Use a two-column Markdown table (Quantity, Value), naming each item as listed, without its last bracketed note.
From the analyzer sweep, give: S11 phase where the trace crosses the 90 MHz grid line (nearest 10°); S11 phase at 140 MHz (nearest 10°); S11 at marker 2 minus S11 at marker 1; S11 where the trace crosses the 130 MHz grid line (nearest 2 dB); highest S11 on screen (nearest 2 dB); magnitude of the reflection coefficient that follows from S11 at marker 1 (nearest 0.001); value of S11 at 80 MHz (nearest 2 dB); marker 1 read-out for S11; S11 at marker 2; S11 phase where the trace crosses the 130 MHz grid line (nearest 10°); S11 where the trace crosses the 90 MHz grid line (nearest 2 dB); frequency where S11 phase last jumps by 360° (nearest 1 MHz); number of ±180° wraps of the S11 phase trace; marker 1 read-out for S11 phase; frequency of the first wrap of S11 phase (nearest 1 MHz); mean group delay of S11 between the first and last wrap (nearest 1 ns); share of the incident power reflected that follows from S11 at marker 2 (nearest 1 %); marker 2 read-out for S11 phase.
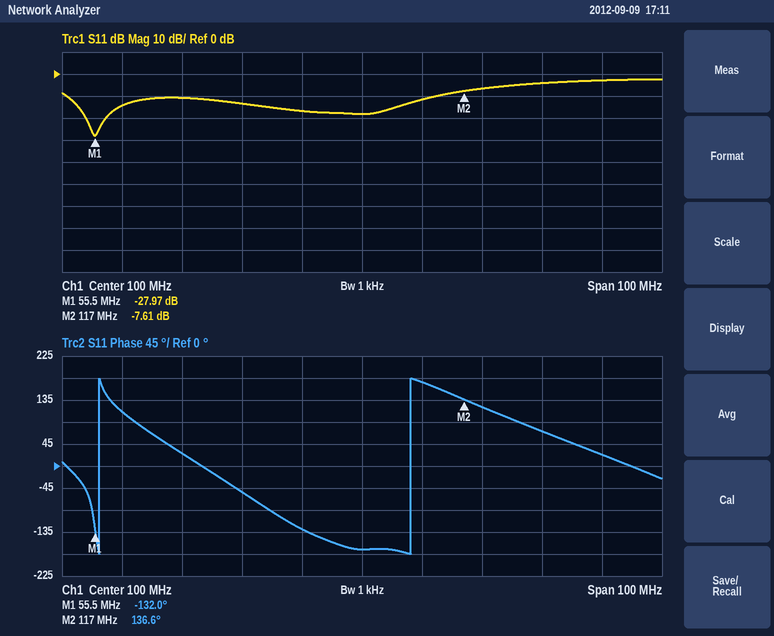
| Quantity | Value |
|---|---|
| S11 phase where the trace crosses the 90 MHz grid line | -130° |
| S11 phase at 140 MHz | 20° |
| S11 at marker 2 minus S11 at marker 1 | 20.36 dB |
| S11 where the trace crosses the 130 MHz grid line | -4 dB |
| highest S11 on screen | -2 dB |
| magnitude of the reflection coefficient that follows from S11 at marker 1 | 0.040 |
| value of S11 at 80 MHz | -14 dB |
| marker 1 read-out for S11 | -27.97 dB |
| S11 at marker 2 | -7.61 dB |
| S11 phase where the trace crosses the 130 MHz grid line | 70° |
| S11 where the trace crosses the 90 MHz grid line | -16 dB |
| frequency where S11 phase last jumps by 360° | 108 MHz |
| number of ±180° wraps of the S11 phase trace | 2 |
| marker 1 read-out for S11 phase | -132.0° |
| frequency of the first wrap of S11 phase | 56 MHz |
| mean group delay of S11 between the first and last wrap | 19 ns |
| share of the incident power reflected that follows from S11 at marker 2 | 17 % |
| marker 2 read-out for S11 phase | 136.6° |
